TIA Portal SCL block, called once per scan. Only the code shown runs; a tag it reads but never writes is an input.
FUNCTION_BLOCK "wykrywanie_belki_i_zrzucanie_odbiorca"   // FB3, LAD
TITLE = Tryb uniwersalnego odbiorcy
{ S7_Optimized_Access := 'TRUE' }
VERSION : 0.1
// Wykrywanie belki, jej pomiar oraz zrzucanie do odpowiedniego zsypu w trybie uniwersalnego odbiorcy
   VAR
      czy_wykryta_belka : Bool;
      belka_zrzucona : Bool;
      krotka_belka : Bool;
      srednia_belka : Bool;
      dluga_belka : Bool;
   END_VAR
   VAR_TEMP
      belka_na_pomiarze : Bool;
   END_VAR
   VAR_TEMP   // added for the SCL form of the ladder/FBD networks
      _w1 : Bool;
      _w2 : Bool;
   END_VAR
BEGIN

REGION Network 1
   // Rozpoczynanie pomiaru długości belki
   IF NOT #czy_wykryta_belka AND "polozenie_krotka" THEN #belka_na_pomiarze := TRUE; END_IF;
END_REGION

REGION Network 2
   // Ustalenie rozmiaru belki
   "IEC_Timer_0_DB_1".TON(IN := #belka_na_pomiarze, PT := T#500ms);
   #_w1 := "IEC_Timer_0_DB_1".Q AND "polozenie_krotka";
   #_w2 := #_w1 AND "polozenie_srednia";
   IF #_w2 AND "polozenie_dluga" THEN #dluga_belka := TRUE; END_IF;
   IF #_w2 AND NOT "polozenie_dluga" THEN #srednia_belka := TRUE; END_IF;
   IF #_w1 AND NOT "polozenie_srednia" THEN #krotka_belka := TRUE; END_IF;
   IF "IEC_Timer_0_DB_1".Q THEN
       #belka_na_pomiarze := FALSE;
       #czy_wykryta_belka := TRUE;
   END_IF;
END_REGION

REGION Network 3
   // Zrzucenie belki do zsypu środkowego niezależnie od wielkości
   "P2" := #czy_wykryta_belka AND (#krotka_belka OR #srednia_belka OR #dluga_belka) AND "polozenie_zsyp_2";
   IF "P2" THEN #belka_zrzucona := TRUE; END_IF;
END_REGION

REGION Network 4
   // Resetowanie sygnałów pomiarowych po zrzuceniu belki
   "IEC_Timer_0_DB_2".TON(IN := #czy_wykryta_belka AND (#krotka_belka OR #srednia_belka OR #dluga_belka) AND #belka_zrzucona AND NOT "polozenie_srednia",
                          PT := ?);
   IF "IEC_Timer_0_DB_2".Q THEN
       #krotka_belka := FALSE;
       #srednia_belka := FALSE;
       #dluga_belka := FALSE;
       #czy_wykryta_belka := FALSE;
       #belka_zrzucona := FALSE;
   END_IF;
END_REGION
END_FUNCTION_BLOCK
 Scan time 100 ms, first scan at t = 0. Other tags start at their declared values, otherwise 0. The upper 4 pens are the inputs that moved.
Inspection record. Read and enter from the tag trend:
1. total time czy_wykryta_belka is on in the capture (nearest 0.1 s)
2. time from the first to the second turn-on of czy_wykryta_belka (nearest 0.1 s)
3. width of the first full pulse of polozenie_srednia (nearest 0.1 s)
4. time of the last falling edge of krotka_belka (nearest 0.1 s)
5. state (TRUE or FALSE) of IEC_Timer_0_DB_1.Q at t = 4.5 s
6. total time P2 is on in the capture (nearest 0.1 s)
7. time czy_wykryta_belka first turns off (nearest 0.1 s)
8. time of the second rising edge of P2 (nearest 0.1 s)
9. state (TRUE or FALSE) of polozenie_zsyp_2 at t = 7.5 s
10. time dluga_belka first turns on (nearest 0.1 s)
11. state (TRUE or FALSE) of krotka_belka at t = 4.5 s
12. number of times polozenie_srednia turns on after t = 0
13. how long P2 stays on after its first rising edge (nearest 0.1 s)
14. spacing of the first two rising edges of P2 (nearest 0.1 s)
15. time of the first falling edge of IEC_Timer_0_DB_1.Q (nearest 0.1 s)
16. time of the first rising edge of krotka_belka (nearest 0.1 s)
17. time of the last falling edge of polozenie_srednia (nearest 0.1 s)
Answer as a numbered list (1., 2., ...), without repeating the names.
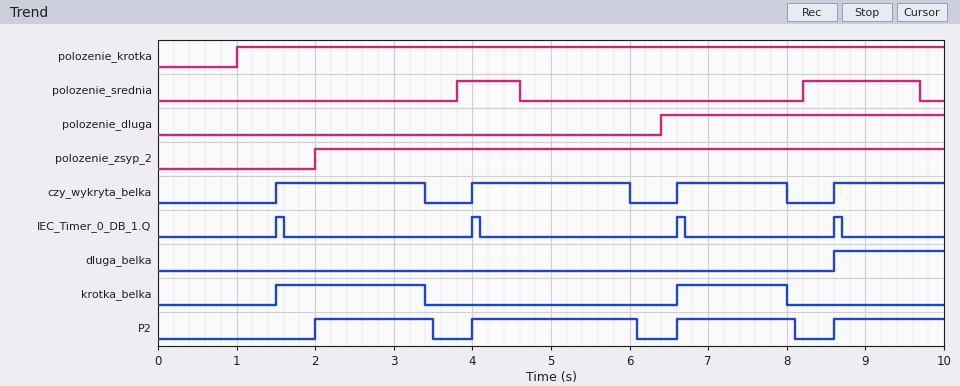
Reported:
1. 6.7 s
2. 2.5 s
3. 0.8 s
4. 8.0 s
5. FALSE
6. 6.5 s
7. 3.4 s
8. 4.0 s
9. TRUE
10. 8.6 s
11. FALSE
12. 2
13. 1.5 s
14. 2.0 s
15. 1.6 s
16. 1.5 s
17. 9.7 s
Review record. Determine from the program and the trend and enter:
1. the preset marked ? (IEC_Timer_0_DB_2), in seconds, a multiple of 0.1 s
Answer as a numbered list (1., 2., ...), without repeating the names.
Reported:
1. 1.4 s
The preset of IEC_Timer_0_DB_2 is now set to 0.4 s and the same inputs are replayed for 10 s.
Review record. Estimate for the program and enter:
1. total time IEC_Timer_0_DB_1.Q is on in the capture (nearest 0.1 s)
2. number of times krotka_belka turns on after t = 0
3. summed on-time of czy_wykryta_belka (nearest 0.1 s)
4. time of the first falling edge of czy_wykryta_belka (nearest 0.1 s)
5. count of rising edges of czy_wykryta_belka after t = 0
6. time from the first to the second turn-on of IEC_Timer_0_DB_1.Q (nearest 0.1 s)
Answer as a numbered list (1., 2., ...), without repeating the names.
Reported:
1. 0.7 s
2. 5
3. 4.9 s
4. 2.4 s
5. 7
6. 1.5 s
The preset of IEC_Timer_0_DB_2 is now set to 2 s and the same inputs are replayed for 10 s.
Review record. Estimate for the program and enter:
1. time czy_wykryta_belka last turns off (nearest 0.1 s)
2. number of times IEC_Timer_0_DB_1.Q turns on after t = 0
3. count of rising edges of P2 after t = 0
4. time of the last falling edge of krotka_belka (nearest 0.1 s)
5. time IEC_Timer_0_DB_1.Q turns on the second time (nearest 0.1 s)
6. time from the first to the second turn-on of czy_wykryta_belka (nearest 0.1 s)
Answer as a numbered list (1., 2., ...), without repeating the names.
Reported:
1. 6.6 s
2. 2
3. 2
4. 6.6 s
5. 7.2 s
6. 5.7 s
